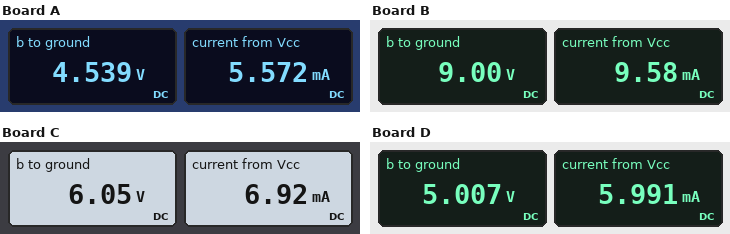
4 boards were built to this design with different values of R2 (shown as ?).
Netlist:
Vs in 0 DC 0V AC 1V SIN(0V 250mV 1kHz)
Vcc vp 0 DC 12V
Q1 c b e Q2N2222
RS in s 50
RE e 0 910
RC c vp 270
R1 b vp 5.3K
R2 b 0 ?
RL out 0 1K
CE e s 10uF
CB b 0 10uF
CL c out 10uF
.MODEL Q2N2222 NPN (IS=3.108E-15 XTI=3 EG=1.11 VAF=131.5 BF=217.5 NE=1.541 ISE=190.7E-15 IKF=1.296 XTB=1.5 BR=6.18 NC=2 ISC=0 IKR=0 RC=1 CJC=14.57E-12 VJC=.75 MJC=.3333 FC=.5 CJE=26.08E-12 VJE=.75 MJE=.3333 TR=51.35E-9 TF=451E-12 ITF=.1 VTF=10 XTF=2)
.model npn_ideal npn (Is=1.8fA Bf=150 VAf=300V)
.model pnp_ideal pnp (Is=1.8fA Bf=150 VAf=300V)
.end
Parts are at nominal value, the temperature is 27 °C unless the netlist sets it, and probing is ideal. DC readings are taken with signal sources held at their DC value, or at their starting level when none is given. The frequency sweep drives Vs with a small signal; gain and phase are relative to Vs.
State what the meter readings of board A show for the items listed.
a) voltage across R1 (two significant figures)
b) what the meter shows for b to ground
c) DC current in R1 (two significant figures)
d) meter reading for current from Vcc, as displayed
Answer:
7.5 V
4.539 V
1.4 mA
5.572 mA
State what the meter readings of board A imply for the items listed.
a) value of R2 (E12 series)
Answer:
3.3 kΩ
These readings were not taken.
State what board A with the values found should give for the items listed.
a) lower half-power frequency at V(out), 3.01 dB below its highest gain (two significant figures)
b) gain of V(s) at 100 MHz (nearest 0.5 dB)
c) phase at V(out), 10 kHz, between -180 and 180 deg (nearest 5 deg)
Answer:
290 Hz
-20.0 dB
0 deg
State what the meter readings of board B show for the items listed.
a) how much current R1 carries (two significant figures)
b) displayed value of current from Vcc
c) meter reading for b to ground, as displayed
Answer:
570 µA
9.58 mA
9.00 V
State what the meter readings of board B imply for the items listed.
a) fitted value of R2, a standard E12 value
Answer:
18 kΩ
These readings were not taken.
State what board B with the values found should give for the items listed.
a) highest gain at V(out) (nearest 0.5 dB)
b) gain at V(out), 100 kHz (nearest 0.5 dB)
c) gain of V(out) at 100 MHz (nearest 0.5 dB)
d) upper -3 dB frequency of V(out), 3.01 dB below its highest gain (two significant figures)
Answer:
12.0 dB
12.0 dB
6.0 dB
59 MHz
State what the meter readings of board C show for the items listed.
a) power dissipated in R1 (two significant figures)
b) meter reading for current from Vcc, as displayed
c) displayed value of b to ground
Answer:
6.7 mW
6.92 mA
6.05 V
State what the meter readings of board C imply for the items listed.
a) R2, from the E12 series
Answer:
5.6 kΩ
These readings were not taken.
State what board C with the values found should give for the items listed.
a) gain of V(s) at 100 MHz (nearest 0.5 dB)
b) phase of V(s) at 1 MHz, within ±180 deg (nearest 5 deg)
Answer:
-22.5 dB
0 deg
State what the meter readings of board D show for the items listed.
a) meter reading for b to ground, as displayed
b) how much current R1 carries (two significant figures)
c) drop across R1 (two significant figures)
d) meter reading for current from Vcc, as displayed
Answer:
5.007 V
1.3 mA
7.0 V
5.991 mA
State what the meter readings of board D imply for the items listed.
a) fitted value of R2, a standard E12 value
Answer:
3.9 kΩ
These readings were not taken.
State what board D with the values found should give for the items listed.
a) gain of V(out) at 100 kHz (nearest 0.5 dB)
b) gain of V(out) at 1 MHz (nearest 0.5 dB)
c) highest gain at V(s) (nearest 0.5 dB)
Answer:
11.5 dB
11.5 dB
0 dB
